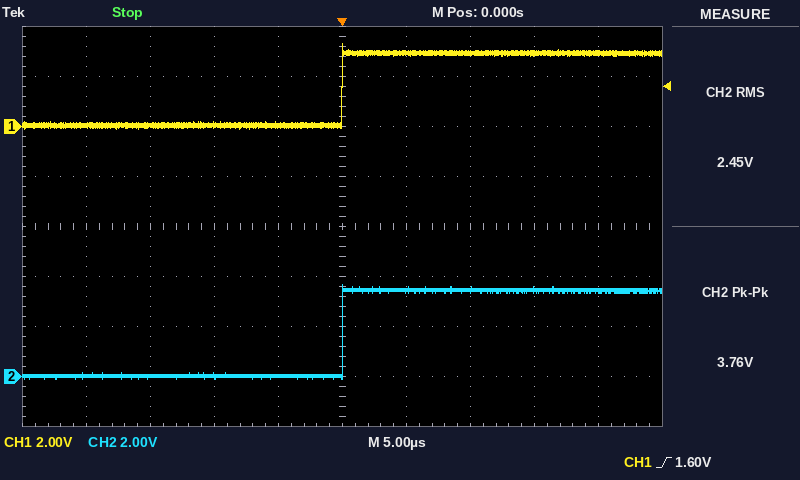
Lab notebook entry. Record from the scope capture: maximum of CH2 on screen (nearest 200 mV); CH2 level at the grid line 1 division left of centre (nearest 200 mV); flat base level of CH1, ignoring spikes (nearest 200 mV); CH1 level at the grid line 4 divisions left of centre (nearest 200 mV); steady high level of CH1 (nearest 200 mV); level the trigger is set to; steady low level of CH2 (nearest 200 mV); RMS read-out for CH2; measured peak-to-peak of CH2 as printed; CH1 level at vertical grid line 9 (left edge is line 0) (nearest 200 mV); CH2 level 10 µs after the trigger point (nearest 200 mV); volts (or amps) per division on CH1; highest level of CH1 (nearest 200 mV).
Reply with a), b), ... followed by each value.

a) 3.6 V
b) 0.0 V
c) 0.0 V
d) 0.0 V
e) 3.0 V
f) 1.60 V
g) 0.0 V
h) 2.45 V
i) 3.76 V
j) 3.0 V
k) 3.4 V
l) 2 V
m) 3.4 V
